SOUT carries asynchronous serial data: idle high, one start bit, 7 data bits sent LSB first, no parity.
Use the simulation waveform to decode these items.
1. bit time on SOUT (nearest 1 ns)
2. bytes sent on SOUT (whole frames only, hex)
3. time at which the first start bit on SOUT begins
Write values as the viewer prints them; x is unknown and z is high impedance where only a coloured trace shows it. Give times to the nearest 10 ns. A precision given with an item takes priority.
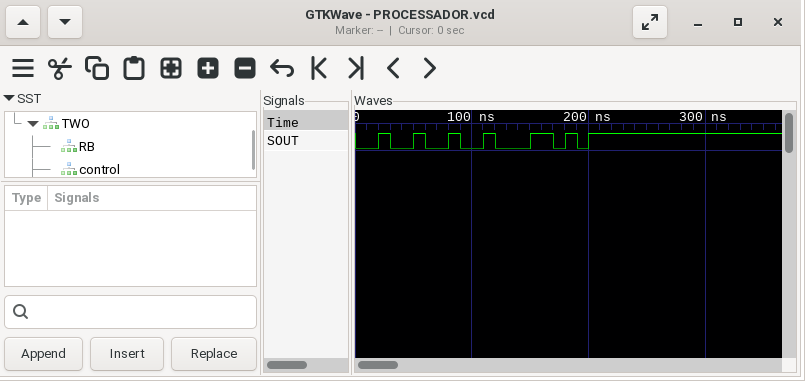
10 ns
12, 2C
30 ns
